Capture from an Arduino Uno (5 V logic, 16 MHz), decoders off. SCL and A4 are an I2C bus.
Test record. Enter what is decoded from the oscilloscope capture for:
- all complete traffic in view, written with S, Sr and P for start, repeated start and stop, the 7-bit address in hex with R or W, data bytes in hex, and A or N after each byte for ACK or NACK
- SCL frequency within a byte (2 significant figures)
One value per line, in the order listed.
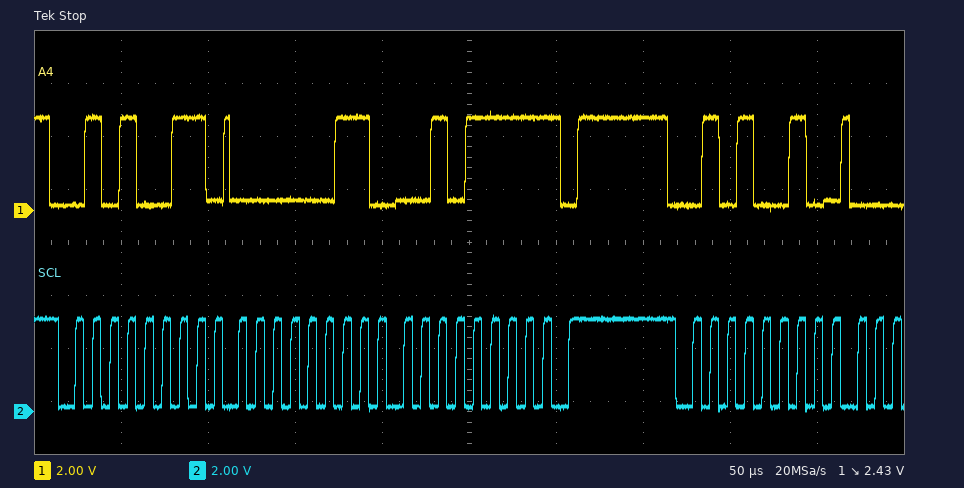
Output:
S 29R A 03 A 2F N P S 29W A
100 kHz
